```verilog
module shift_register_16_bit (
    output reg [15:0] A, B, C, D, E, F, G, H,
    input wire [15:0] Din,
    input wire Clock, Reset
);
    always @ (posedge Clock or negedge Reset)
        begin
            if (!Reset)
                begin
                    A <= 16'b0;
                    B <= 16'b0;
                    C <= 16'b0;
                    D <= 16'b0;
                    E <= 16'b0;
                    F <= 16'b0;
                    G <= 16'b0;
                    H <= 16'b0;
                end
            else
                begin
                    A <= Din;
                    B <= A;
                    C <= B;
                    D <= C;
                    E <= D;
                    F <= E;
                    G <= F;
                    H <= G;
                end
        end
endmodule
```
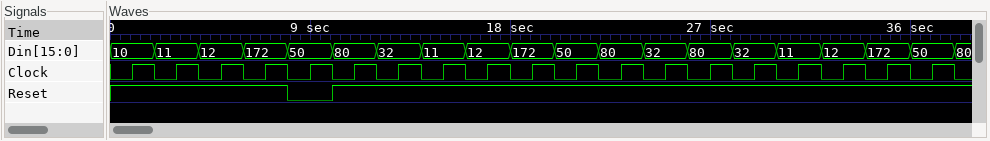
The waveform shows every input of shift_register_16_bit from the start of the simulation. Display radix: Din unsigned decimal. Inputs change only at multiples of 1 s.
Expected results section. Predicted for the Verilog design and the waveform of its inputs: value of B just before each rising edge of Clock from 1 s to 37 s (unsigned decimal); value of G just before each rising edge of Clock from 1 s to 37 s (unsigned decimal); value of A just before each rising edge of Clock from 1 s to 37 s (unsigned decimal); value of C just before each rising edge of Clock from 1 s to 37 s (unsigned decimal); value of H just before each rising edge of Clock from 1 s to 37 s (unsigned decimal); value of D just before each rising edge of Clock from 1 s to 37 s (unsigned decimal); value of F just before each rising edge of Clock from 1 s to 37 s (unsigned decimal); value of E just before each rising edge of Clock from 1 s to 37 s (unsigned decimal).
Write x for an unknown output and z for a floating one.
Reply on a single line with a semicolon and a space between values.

x, x, 10, 11, 0, 0, 0, 80, 32, 11, 12, 172, 50, 80, 32, 80, 32, 11, 12; x, x, x, x, 0, 0, 0, 0, 0, 0, 0, 0, 80, 32, 11, 12, 172, 50, 80; x, 10, 11, 12, 0, 0, 80, 32, 11, 12, 172, 50, 80, 32, 80, 32, 11, 12, 172; x, x, x, 10, 0, 0, 0, 0, 80, 32, 11, 12, 172, 50, 80, 32, 80, 32, 11; x, x, x, x, 0, 0, 0, 0, 0, 0, 0, 0, 0, 80, 32, 11, 12, 172, 50; x, x, x, x, 0, 0, 0, 0, 0, 80, 32, 11, 12, 172, 50, 80, 32, 80, 32; x, x, x, x, 0, 0, 0, 0, 0, 0, 0, 80, 32, 11, 12, 172, 50, 80, 32; x, x, x, x, 0, 0, 0, 0, 0, 0, 80, 32, 11, 12, 172, 50, 80, 32, 80
